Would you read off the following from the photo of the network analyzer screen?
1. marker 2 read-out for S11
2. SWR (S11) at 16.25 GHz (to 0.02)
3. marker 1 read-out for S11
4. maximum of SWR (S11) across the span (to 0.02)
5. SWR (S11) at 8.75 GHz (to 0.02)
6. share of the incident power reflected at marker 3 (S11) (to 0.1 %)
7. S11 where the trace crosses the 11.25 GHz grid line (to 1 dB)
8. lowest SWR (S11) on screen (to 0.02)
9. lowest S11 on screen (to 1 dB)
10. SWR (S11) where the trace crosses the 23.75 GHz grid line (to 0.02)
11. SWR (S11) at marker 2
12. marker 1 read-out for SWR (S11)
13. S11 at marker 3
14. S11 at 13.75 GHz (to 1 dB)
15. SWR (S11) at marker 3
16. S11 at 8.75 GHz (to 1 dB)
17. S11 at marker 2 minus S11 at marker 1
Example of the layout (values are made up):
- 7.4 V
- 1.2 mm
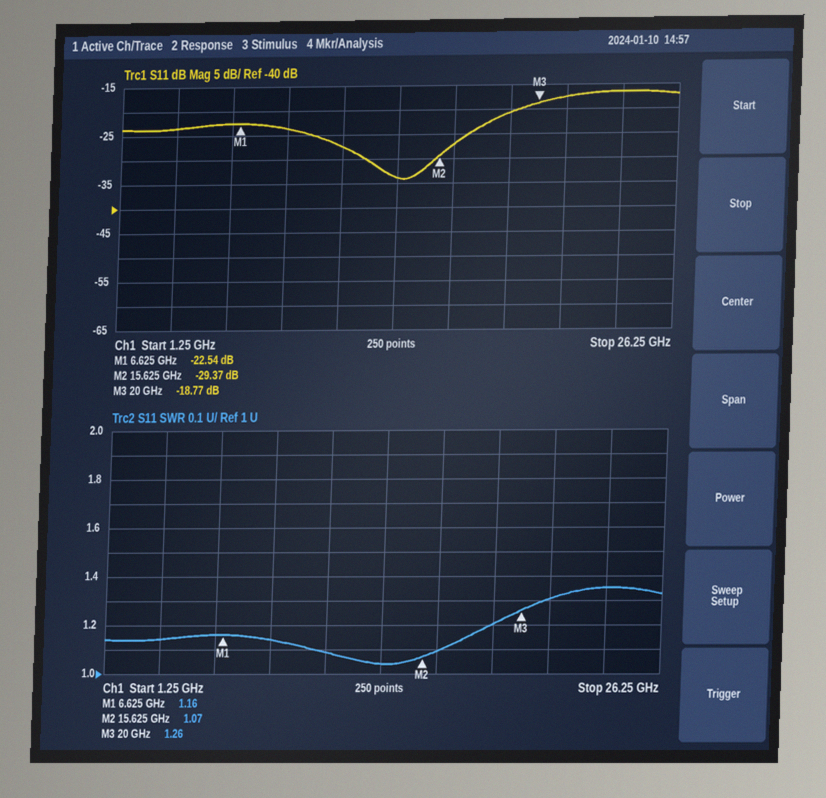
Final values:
- -29.37 dB
- 1.10
- -22.54 dB
- 1.36
- 1.14
- 1.3 %
- -27 dB
- 1.04
- -34 dB
- 1.36
- 1.07
- 1.16
- -18.77 dB
- -34 dB
- 1.26
- -24 dB
- -6.83 dB
